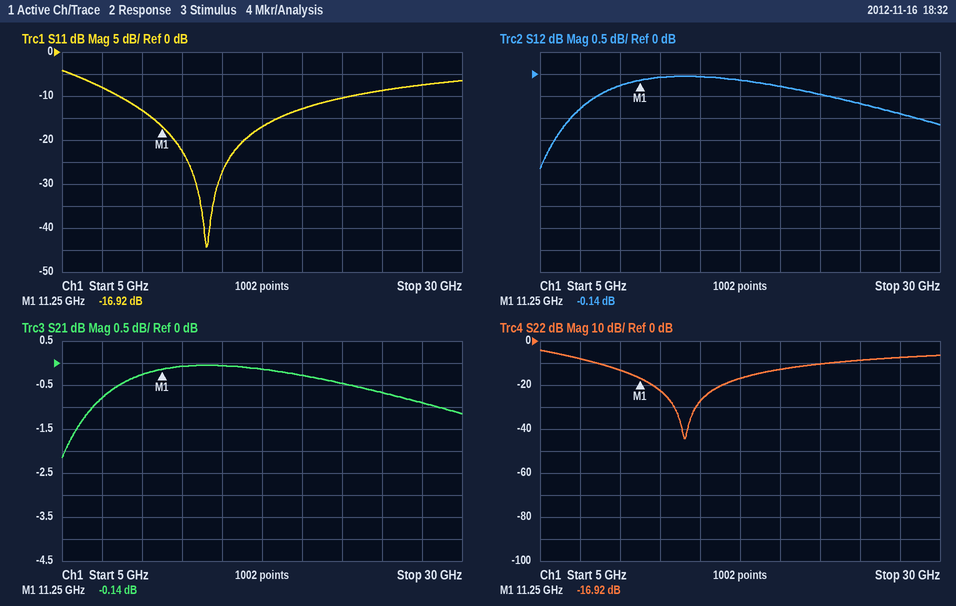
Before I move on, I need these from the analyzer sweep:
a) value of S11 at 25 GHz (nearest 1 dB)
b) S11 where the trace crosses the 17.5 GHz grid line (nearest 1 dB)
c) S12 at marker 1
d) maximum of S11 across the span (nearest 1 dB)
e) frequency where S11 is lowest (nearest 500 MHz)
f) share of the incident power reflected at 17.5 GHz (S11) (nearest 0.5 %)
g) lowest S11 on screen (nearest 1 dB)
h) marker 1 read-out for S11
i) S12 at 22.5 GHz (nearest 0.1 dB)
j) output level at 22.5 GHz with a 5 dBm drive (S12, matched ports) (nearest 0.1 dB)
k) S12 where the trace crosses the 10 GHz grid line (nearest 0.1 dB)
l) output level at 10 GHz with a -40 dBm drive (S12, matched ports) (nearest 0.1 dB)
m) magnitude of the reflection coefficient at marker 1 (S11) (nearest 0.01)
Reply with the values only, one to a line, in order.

-9 dB
-17 dB
-0.14 dB
-4 dB
14.0 GHz
2.0 %
-44 dB
-16.92 dB
-0.5 dB
4.5 dBm
-0.3 dB
-40.3 dBm
0.14
